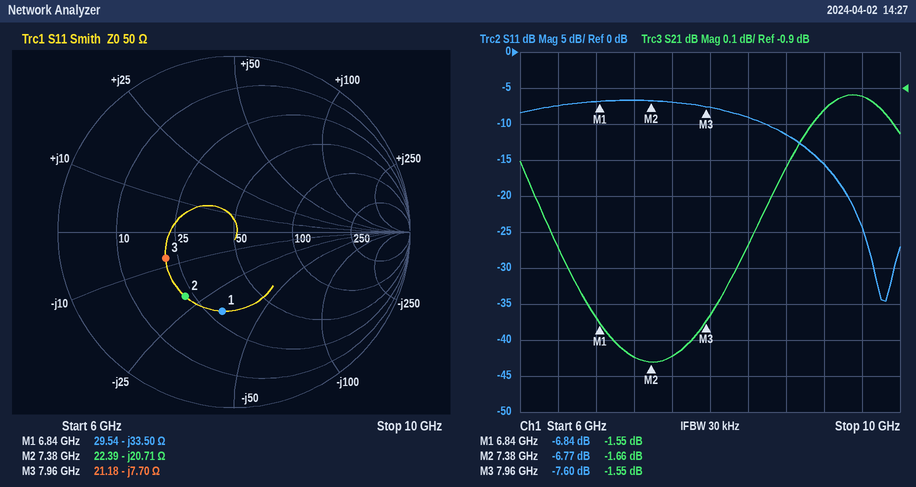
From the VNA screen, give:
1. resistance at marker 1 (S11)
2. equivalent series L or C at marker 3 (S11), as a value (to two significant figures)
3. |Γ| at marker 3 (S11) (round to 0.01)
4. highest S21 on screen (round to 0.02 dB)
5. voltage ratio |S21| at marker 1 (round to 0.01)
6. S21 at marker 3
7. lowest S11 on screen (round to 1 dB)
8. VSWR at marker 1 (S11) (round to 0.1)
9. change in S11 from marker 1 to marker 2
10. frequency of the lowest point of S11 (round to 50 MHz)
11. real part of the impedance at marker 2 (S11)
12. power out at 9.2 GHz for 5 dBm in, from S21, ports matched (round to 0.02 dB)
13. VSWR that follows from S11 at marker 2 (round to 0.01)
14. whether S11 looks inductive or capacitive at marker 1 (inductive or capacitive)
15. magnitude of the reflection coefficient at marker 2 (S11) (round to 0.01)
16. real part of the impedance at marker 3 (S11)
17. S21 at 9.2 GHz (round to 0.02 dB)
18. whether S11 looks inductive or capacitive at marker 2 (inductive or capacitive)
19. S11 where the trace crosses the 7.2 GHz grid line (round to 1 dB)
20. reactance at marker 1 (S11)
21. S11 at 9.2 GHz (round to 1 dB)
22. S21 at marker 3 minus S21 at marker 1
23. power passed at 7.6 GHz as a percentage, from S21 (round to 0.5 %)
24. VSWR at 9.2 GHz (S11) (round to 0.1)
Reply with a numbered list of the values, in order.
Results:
1. 29.54 Ω
2. 2.6 pF
3. 0.42
4. -0.92 dB
5. 0.84
6. -1.55 dB
7. -35 dB
8. 2.7
9. 0.07 dB
10. 9.85 GHz
11. 22.39 Ω
12. 4.04 dBm
13. 2.69
14. capacitive
15. 0.46
16. 21.18 Ω
17. -0.96 dB
18. capacitive
19. -7 dB
20. -33.50 Ω
21. -16 dB
22. 0.00 dB
23. 68.5 %
24. 1.4
